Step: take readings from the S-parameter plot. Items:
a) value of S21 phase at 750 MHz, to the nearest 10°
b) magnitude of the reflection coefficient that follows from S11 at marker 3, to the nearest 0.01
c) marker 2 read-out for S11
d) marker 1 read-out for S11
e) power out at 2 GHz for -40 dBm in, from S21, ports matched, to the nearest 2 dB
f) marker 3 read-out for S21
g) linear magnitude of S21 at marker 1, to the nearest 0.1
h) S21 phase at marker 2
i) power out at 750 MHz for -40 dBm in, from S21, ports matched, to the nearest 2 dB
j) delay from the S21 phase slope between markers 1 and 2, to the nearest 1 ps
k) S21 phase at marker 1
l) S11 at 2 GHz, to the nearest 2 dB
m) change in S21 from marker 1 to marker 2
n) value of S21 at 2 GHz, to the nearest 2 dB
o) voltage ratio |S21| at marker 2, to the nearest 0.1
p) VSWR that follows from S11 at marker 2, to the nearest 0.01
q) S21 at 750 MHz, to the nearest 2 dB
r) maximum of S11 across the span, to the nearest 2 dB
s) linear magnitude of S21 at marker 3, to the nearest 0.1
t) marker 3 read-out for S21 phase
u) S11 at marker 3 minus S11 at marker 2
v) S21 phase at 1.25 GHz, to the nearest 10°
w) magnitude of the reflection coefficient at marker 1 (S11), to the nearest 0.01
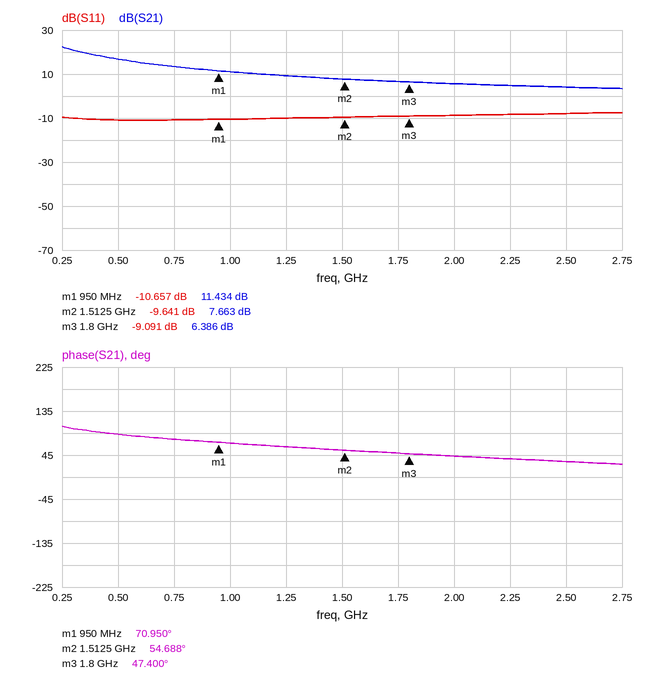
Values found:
80°
0.35
-9.641 dB
-10.657 dB
-34 dBm
6.386 dB
3.7
54.688°
-26 dBm
80 ps
70.950°
-8 dB
-3.771 dB
6 dB
2.4
1.98
14 dB
-8 dB
2.1
47.400°
0.550 dB
60°
0.29
